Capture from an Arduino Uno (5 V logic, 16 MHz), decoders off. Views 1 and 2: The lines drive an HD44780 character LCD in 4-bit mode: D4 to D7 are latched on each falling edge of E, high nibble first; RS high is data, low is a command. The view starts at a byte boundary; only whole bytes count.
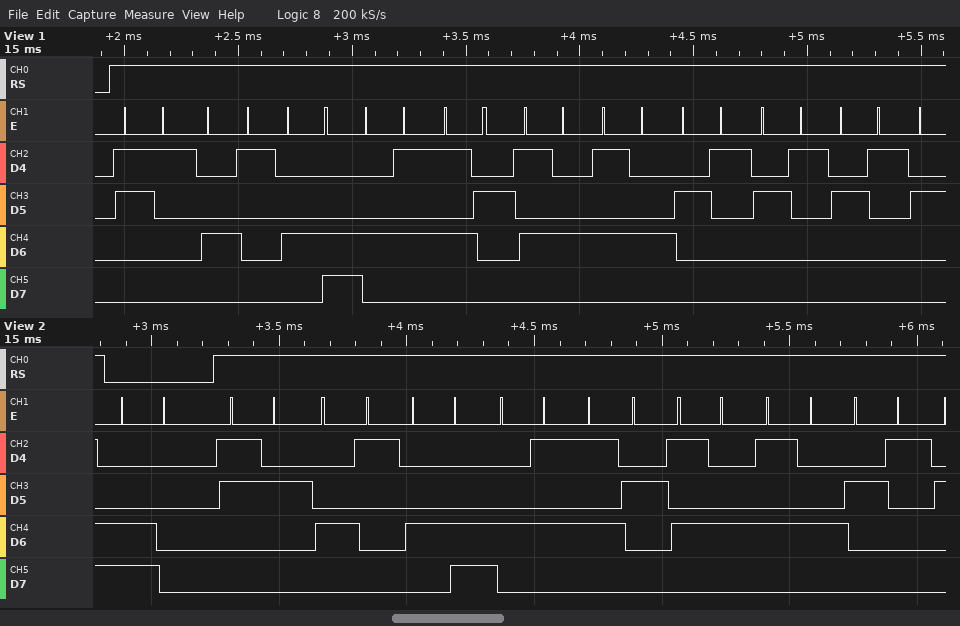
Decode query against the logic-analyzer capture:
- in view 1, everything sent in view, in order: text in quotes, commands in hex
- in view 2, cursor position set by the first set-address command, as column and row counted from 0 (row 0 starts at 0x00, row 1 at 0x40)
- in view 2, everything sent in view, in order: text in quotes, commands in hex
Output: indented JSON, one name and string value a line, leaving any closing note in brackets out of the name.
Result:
{
  "in view 1, everything sent in view, in order: text in quotes, commands in hex": "\"1ALERTT!!!\"",
  "in view 2, cursor position set by the first set-address command, as column and row counted from 0": "column 0, row 1",
  "in view 2, everything sent in view, in order: text in quotes, commands in hex": "0xC0 \"2ALERTT!\""
}
